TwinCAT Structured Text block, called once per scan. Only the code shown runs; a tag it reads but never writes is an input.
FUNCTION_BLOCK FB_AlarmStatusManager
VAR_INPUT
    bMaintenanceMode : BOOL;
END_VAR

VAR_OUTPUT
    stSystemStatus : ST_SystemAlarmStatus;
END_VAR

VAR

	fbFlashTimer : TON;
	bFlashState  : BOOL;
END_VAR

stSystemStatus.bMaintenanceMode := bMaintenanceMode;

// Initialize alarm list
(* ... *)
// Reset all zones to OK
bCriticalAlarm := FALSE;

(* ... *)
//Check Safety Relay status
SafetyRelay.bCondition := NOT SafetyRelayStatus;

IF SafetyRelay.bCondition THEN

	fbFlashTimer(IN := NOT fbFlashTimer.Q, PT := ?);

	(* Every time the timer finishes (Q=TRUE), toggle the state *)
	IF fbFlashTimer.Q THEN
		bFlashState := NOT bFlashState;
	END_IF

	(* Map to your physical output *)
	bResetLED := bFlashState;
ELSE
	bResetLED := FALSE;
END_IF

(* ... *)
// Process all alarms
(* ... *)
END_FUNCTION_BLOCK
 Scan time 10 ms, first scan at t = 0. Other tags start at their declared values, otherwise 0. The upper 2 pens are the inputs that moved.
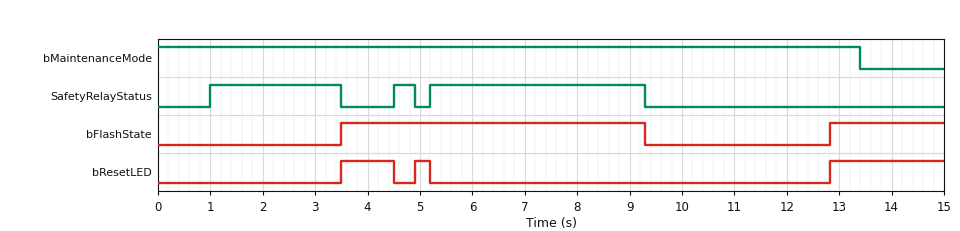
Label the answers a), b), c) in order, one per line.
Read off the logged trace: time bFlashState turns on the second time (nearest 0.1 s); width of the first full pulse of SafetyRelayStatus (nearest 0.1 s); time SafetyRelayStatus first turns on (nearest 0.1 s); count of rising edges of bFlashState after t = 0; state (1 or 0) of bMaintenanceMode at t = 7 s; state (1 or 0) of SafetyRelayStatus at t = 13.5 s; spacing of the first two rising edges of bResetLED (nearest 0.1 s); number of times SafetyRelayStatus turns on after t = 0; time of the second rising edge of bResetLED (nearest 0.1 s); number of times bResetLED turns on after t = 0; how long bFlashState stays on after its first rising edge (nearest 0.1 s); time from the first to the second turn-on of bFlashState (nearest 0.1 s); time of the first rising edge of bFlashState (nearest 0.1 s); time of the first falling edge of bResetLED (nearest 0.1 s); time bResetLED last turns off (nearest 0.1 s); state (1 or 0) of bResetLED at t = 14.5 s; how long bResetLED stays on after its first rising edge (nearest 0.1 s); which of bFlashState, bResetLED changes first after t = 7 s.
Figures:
a) 12.8 s
b) 2.5 s
c) 1.0 s
d) 2
e) 1
f) 0
g) 1.4 s
h) 3
i) 4.9 s
j) 3
k) 5.8 s
l) 9.3 s
m) 3.5 s
n) 4.5 s
o) 5.2 s
p) 1
q) 1.0 s
r) bFlashState
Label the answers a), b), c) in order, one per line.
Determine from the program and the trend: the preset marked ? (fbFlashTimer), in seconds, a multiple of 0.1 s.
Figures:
a) 3.5 s
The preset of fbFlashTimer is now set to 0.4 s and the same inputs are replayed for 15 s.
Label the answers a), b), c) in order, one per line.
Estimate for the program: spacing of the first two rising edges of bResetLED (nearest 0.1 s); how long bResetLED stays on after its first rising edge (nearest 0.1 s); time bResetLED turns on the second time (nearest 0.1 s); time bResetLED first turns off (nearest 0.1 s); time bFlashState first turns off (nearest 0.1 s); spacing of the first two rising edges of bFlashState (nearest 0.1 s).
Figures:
a) 3.1 s
b) 0.4 s
c) 3.5 s
d) 0.8 s
e) 0.8 s
f) 3.1 s
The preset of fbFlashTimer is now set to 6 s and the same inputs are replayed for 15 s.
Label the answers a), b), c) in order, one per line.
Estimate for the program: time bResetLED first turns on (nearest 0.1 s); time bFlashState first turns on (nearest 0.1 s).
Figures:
a) 9.3 s
b) 9.3 s
